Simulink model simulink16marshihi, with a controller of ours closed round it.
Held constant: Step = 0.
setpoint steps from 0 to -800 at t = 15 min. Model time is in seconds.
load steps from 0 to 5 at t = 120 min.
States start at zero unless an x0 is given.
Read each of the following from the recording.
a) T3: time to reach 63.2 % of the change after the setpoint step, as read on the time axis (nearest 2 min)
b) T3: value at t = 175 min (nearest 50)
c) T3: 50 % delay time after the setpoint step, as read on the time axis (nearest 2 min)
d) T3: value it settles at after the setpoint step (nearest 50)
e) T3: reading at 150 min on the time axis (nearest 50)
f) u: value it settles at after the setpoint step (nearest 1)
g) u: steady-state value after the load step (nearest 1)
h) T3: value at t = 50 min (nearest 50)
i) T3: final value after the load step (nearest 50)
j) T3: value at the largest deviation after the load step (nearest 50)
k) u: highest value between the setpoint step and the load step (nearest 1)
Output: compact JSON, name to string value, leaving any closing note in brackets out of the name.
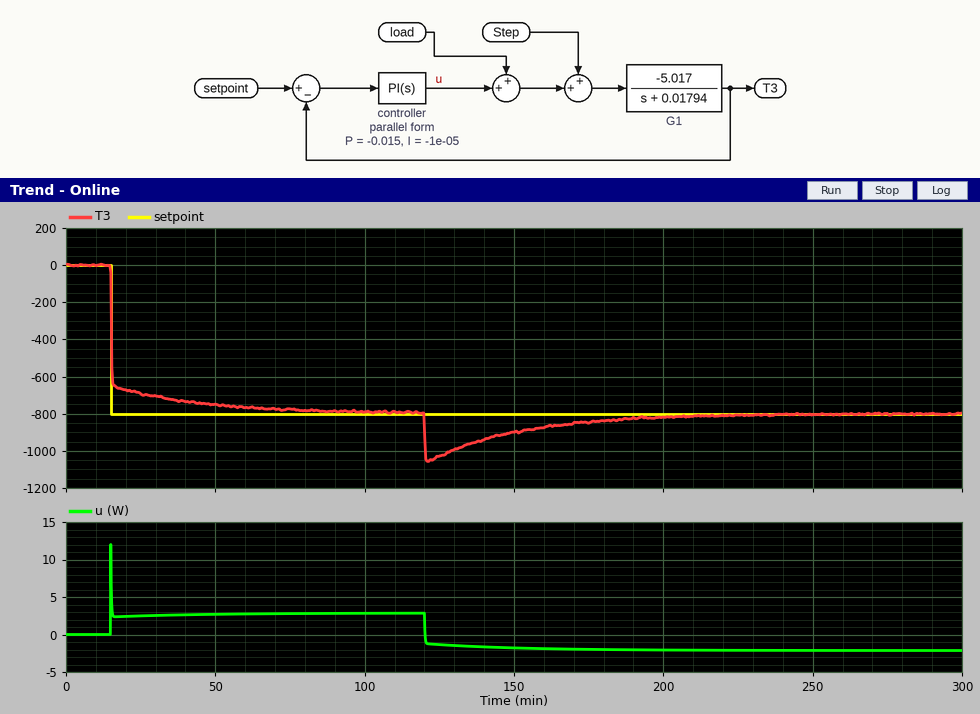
{"T3: time to reach 63.2 % of the change after the setpoint step, as read on the time axis": "16 min", "T3: value at t = 175 min": "-850", "T3: 50 % delay time after the setpoint step, as read on the time axis": "16 min", "T3: value it settles at after the setpoint step": "-800", "T3: reading at 150 min on the time axis": "-900", "u: value it settles at after the setpoint step": "3", "u: steady-state value after the load step": "-2", "T3: value at t = 50 min": "-750", "T3: final value after the load step": "-800", "T3: value at the largest deviation after the load step": "-1050", "u: highest value between the setpoint step and the load step": "12"}
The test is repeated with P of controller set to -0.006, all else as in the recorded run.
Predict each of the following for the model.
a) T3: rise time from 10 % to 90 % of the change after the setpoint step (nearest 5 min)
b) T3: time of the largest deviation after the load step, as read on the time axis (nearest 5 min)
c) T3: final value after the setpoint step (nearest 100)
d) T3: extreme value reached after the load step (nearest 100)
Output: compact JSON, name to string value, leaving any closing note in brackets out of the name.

{"T3: rise time from 10 % to 90 % of the change after the setpoint step": "20 min", "T3: time of the largest deviation after the load step, as read on the time axis": "120 min", "T3: final value after the setpoint step": "-800", "T3: extreme value reached after the load step": "-1300"}
